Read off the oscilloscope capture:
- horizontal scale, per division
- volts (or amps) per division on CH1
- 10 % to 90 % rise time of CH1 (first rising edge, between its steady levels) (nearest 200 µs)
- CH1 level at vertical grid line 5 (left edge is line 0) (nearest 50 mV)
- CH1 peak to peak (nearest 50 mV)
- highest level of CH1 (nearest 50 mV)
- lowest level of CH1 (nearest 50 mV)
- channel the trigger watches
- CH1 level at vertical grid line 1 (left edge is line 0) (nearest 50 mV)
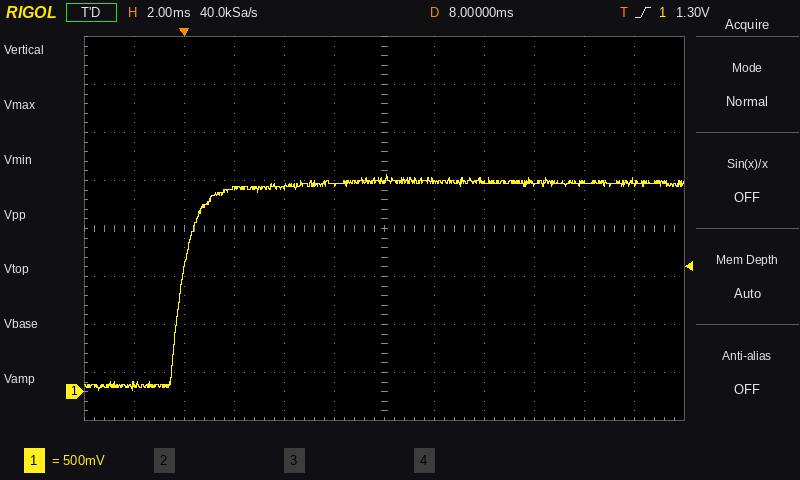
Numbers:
2 ms
500 mV
1.4 ms
2.15 V
2.25 V
2.25 V
0 mV
CH1
50 mV
